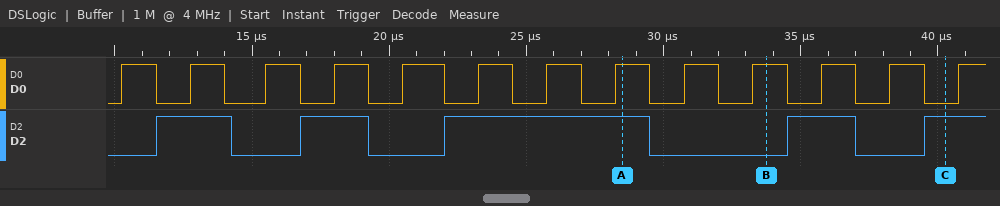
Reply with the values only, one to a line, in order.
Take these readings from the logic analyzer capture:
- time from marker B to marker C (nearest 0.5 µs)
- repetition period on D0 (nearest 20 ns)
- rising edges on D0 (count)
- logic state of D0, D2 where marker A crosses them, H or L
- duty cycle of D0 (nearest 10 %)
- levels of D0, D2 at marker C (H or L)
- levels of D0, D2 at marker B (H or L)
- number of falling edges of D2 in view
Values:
6.5 µs
2540 ns
13
D0=H, D2=H
50 %
D0=L, D2=H
D0=H, D2=L
4
